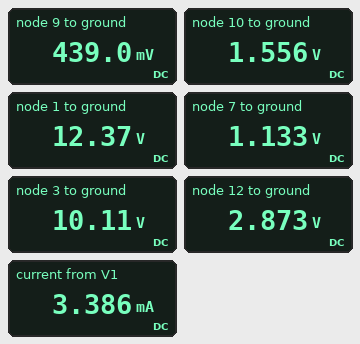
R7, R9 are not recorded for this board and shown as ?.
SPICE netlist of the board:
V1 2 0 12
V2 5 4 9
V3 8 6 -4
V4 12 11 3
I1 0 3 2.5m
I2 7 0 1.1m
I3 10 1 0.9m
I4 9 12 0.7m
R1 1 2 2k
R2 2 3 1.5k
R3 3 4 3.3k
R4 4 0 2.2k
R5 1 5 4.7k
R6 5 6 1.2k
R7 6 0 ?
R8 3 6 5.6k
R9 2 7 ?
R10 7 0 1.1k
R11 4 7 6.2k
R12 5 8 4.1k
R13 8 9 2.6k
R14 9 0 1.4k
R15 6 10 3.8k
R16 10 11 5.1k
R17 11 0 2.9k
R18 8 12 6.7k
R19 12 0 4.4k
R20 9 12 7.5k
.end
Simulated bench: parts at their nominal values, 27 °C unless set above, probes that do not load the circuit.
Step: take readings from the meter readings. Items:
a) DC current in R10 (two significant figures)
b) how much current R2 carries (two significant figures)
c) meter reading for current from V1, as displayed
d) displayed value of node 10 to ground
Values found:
1.0 mA
1.3 mA
3.386 mA
1.556 V
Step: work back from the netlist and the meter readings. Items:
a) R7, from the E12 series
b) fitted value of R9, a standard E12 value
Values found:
2.2 kΩ
4.7 kΩ
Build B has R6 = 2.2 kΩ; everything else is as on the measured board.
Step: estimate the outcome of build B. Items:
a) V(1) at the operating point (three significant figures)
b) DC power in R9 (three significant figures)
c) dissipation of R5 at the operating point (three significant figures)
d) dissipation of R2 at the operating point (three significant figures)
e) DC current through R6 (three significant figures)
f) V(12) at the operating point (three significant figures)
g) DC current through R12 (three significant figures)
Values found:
12.5 V
24.9 mW
1.98 mW
2.24 mW
1.65 mA
2.74 V
1.86 mA
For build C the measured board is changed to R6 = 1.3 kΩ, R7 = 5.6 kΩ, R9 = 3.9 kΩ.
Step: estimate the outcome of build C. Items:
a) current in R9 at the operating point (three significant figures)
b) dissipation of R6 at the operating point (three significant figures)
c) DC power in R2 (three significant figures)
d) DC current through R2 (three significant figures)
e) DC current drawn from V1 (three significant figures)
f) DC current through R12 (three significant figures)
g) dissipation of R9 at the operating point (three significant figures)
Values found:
2.67 mA
3.88 mW
1.39 mW
963 µA
3.32 mA
1.52 mA
27.8 mW
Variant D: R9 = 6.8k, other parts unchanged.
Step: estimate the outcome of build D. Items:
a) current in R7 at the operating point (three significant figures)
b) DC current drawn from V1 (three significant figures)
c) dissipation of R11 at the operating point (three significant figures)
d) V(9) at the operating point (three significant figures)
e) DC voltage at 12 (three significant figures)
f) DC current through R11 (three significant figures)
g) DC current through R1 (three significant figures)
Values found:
2.82 mA
2.78 mA
58.2 µW
427 mV
2.86 V
96.9 µA
174 µA
